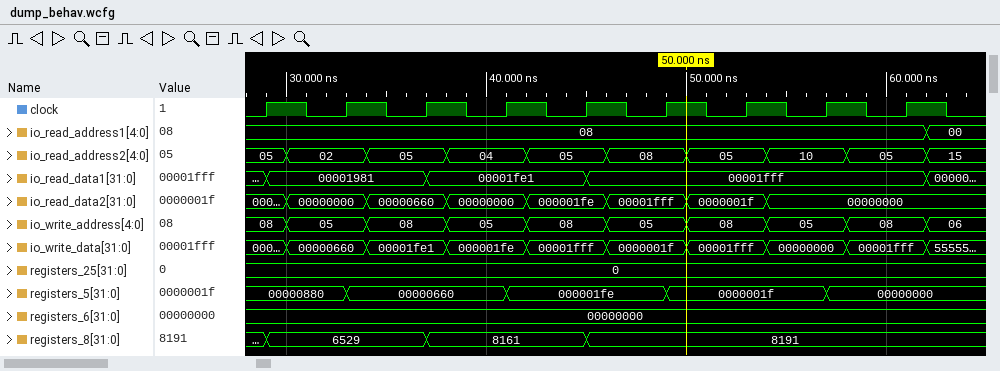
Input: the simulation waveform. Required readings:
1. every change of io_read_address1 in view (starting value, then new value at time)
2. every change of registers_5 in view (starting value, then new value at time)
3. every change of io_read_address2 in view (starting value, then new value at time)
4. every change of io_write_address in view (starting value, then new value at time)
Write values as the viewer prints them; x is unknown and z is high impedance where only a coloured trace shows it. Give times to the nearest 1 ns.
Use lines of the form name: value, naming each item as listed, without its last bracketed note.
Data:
every change of io_read_address1 in view: 08, 00 at 62 ns
every change of registers_5 in view: 00000880, 00000660 at 33 ns, 000001fe at 41 ns, 0000001f at 49 ns, 00000000 at 57 ns
every change of io_read_address2 in view: 05, 02 at 30 ns, 05 at 34 ns, 04 at 38 ns, 05 at 42 ns, 08 at 46 ns, 05 at 50 ns, 10 at 54 ns, 05 at 58 ns, 15 at 62 ns
every change of io_write_address in view: 08, 05 at 30 ns, 08 at 34 ns, 05 at 38 ns, 08 at 42 ns, 05 at 46 ns, 08 at 50 ns, 05 at 54 ns, 08 at 58 ns, 06 at 62 ns
